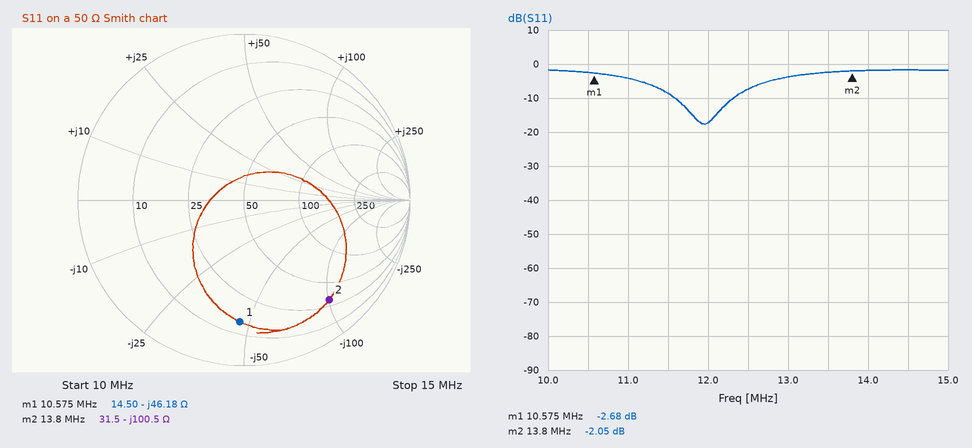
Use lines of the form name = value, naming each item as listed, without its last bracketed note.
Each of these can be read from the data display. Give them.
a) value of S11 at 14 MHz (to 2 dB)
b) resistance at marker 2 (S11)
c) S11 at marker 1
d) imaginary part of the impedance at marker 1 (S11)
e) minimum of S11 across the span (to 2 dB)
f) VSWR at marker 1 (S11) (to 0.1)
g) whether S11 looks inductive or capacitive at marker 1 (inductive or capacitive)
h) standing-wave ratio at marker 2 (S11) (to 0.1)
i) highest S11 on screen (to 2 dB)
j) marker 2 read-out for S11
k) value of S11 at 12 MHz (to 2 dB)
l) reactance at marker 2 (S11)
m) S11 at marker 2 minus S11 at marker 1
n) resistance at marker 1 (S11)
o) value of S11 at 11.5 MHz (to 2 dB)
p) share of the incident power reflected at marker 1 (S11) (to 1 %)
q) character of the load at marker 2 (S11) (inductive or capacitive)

value of S11 at 14 MHz = -2 dB
resistance at marker 2 = 31.5 Ω
S11 at marker 1 = -2.68 dB
imaginary part of the impedance at marker 1 = -46.18 Ω
minimum of S11 across the span = -18 dB
VSWR at marker 1 (S11) = 6.5
whether S11 looks inductive or capacitive at marker 1 = capacitive
standing-wave ratio at marker 2 (S11) = 8.5
highest S11 on screen = -2 dB
marker 2 read-out for S11 = -2.05 dB
value of S11 at 12 MHz = -18 dB
reactance at marker 2 = -100.5 Ω
S11 at marker 2 minus S11 at marker 1 = 0.63 dB
resistance at marker 1 = 14.50 Ω
value of S11 at 11.5 MHz = -8 dB
share of the incident power reflected at marker 1 (S11) = 54 %
character of the load at marker 2 (S11) = capacitive
